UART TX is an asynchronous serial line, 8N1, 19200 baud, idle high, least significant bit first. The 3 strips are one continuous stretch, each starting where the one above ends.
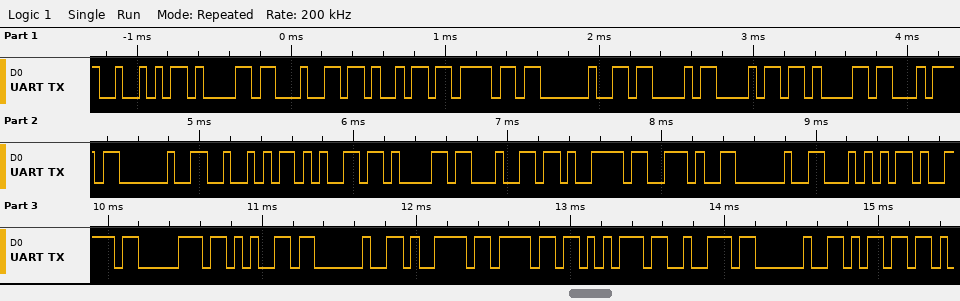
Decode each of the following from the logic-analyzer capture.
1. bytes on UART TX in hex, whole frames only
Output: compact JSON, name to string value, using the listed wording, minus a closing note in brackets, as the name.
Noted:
{"bytes on UART TX in hex, whole frames only": "52 61 64 69 6F 20 43 68 61 74 20 52 65 61 64 79 2E 20 54 79 70 65 20 79 6F 75 72 20 6D"}
